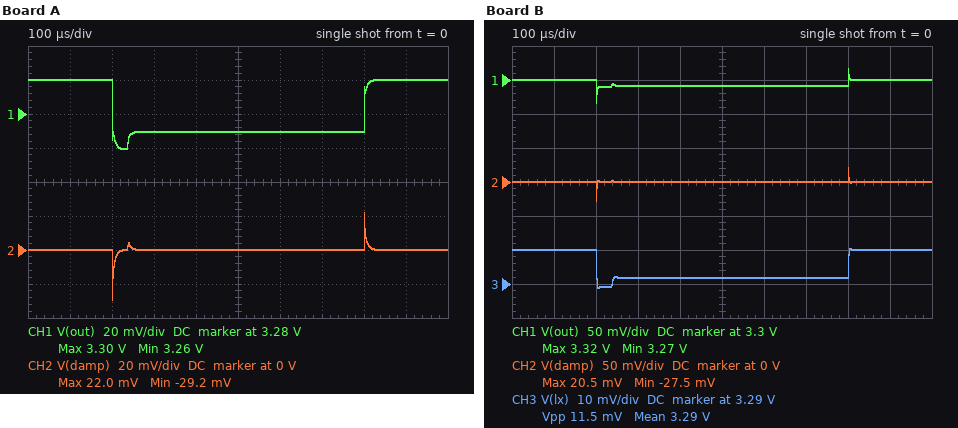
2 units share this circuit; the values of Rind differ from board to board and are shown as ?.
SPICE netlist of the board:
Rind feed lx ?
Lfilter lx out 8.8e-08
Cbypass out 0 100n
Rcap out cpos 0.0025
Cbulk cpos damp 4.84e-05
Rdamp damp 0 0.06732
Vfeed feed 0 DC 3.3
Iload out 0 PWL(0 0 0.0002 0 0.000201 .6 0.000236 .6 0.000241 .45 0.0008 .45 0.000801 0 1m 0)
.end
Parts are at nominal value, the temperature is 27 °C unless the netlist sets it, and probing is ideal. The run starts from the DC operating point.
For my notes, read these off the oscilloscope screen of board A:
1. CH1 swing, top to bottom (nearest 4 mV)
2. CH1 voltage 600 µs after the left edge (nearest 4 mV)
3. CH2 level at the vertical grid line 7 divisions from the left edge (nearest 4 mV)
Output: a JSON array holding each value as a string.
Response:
["40 mV", "3.268 V", "0 V"]
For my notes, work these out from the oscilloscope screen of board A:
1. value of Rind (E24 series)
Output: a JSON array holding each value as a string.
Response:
["0.068 Ω"]
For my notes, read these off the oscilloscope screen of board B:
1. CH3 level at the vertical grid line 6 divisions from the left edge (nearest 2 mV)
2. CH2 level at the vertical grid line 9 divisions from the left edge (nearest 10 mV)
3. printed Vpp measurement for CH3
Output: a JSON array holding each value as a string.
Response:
["3.292 V", "0 V", "11.5 mV"]
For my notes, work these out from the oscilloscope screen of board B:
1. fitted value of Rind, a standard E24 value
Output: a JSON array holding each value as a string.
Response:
["0.018 Ω"]
